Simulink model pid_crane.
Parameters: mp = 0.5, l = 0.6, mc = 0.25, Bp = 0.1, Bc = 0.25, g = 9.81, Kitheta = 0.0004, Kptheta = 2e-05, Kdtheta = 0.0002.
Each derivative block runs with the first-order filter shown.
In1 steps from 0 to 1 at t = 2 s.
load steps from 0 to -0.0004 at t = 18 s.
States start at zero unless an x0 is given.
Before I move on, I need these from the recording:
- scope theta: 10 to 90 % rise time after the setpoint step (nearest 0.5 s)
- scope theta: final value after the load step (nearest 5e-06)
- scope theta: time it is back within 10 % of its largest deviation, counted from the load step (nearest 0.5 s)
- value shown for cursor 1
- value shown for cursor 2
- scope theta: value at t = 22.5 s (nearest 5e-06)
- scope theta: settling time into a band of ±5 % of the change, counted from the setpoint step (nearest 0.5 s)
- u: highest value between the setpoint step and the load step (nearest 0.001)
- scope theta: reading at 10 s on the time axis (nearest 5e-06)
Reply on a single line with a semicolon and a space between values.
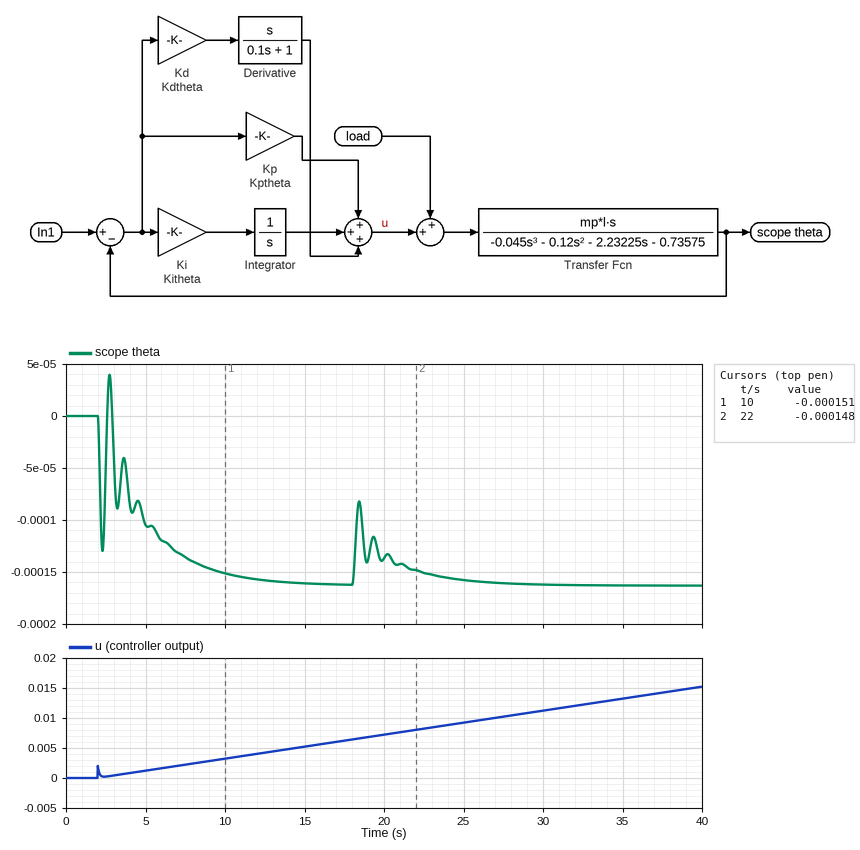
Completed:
7.0 s; -0.000165; 6.0 s; -0.000151; -0.000148; -0.000150; 9.0 s; 0.006; -0.000150
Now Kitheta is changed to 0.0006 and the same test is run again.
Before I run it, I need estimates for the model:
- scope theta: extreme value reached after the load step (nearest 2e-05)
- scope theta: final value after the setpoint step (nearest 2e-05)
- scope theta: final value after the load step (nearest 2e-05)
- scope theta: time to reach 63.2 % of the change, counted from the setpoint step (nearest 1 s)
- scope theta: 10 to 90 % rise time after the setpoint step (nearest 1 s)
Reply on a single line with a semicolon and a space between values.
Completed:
-0.00016; -0.00024; -0.00024; 3 s; 7 s
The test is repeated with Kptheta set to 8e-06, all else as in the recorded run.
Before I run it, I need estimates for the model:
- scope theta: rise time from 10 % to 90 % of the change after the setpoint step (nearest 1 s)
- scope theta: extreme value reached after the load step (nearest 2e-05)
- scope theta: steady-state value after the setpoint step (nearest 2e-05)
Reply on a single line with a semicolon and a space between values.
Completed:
7 s; -0.00008; -0.00016
